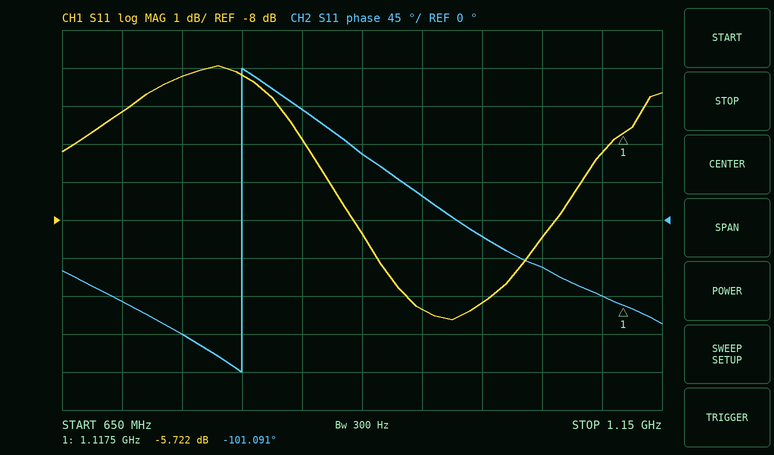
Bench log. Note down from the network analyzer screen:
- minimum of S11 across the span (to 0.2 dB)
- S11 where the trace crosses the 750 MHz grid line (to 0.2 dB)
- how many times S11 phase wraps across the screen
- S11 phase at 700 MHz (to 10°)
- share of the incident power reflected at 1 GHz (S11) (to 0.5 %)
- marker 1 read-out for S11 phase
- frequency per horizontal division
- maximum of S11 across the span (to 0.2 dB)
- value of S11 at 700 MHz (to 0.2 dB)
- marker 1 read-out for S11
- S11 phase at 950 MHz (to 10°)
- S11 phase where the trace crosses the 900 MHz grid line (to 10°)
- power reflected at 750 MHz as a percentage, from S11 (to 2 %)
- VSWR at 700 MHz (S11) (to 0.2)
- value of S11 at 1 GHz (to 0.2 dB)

-10.6 dB
-4.2 dB
1
-100°
9.5 %
-101.091°
50 MHz
-4.0 dB
-5.2 dB
-5.722 dB
30°
80°
38 %
3.4
-10.2 dB
